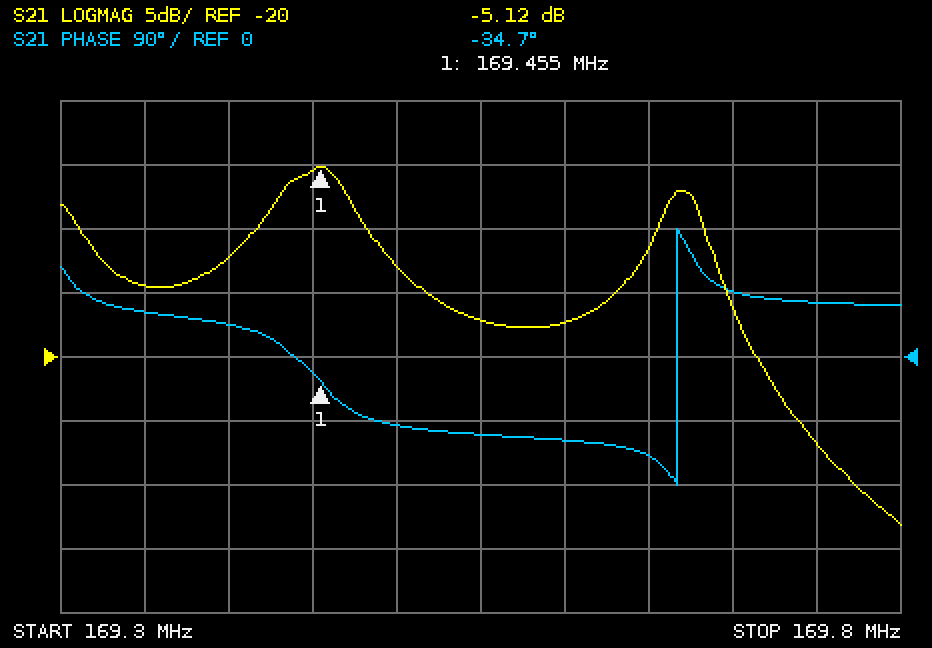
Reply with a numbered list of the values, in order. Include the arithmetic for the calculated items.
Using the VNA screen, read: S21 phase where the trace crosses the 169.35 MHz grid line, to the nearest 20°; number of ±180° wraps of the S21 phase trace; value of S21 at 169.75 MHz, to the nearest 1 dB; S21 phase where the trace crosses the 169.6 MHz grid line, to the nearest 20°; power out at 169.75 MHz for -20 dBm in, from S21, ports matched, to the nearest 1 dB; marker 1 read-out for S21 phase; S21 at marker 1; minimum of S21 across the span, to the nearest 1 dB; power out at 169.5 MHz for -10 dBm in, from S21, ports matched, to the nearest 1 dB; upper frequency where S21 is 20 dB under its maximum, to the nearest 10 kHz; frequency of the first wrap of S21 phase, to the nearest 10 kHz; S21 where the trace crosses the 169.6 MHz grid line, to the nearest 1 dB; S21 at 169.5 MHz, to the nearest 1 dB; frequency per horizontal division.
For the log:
1. 60°
2. 1
3. -27 dB
4. -120°
5. -20 dBm + (-27 dB) = -47 dBm
6. -34.7°
7. -5.12 dB
8. -33 dB
9. -10 dBm + (-13 dB) = -23 dBm
10. 169.74 MHz
11. 169.67 MHz
12. -17 dB
13. -13 dB
14. 50 kHz
